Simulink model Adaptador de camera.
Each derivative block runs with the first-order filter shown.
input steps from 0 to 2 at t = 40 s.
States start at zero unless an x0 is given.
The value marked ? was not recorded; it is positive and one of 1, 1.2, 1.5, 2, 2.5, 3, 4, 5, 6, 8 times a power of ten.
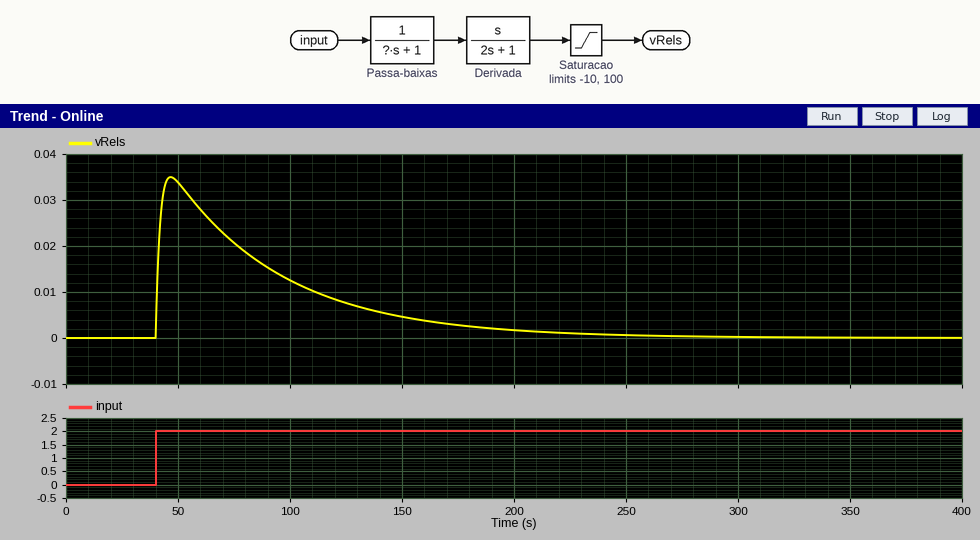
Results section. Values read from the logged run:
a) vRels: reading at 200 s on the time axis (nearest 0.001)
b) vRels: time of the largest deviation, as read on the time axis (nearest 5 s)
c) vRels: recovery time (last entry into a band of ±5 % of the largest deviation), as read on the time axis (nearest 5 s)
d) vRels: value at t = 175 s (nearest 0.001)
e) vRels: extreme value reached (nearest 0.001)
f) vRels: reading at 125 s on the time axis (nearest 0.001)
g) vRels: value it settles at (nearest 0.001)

0.002
45 s
200 s
0.003
0.035
0.008
0.000
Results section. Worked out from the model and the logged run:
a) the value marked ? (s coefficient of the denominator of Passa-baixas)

50
